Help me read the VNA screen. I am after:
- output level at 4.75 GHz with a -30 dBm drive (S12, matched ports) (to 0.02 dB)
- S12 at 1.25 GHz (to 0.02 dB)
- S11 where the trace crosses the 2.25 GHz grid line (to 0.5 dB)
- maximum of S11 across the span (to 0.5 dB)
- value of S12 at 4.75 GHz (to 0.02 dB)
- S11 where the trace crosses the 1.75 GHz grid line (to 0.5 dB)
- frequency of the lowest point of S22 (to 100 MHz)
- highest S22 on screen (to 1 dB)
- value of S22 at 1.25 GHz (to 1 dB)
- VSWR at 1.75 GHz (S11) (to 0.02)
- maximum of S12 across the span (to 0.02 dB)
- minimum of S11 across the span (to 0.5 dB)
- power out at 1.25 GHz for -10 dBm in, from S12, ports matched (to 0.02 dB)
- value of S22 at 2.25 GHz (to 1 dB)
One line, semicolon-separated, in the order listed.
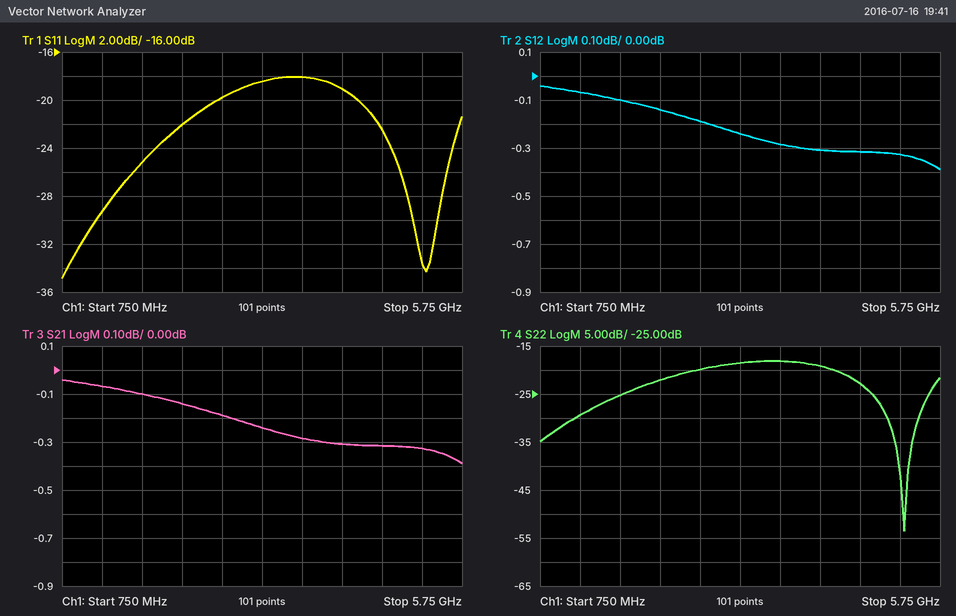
-30.32 dBm; -0.06 dB; -22.0 dB; -18.0 dB; -0.32 dB; -25.0 dB; 5.3 GHz; -18 dB; -29 dB; 1.12; -0.04 dB; -35.0 dB; -10.06 dBm; -22 dB
